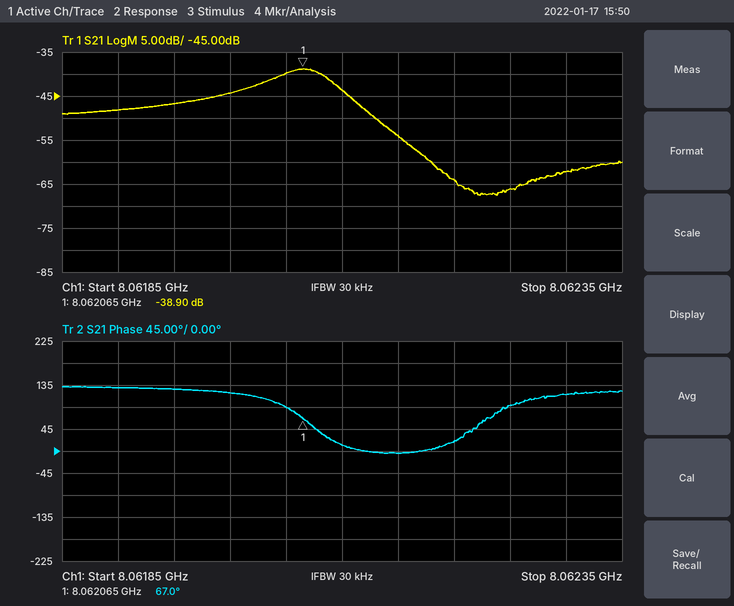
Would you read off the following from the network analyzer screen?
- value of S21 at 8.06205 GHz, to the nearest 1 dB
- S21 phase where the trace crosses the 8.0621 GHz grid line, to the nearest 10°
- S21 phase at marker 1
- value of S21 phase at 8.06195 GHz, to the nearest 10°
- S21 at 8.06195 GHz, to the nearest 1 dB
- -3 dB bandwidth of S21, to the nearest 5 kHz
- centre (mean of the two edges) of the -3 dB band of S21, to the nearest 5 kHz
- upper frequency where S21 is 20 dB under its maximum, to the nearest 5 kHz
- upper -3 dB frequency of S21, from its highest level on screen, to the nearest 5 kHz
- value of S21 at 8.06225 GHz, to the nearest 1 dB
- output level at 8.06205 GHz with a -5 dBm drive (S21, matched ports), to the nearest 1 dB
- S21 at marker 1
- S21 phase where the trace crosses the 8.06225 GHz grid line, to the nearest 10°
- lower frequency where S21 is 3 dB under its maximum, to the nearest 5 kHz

-40 dB
10°
67.0°
130°
-47 dB
60 kHz
8.062060 GHz
8.062175 GHz
8.062090 GHz
-66 dB
-45 dBm
-38.90 dB
90°
8.062030 GHz
